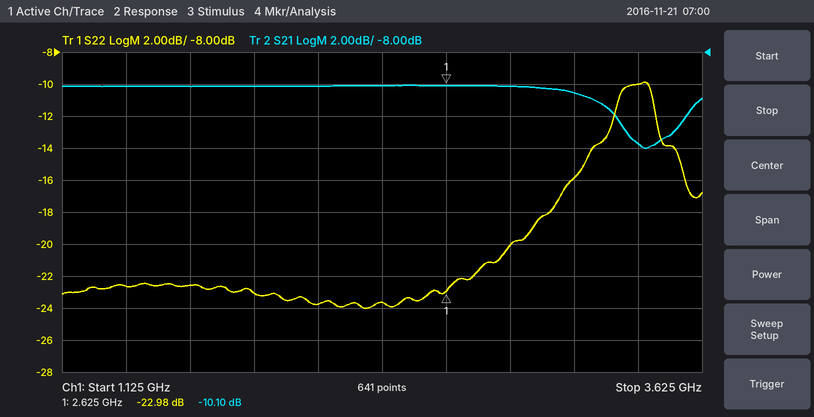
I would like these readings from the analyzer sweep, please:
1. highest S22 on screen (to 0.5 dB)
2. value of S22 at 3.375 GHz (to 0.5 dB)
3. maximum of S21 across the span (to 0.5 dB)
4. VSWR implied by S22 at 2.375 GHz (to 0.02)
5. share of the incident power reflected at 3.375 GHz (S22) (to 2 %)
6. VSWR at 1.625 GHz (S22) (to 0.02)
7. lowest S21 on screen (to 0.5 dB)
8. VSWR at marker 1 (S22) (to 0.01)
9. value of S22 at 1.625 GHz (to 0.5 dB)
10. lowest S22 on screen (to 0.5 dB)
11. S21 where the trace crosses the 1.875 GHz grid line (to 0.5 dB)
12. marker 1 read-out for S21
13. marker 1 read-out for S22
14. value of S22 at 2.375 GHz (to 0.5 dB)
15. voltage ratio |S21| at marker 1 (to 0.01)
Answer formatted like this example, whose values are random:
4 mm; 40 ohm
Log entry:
-10.0 dB; -10.0 dB; -10.0 dB; 1.14; 10 %; 1.16; -14.0 dB; 1.15; -22.5 dB; -24.0 dB; -10.0 dB; -10.10 dB; -22.98 dB; -23.5 dB; 0.31
